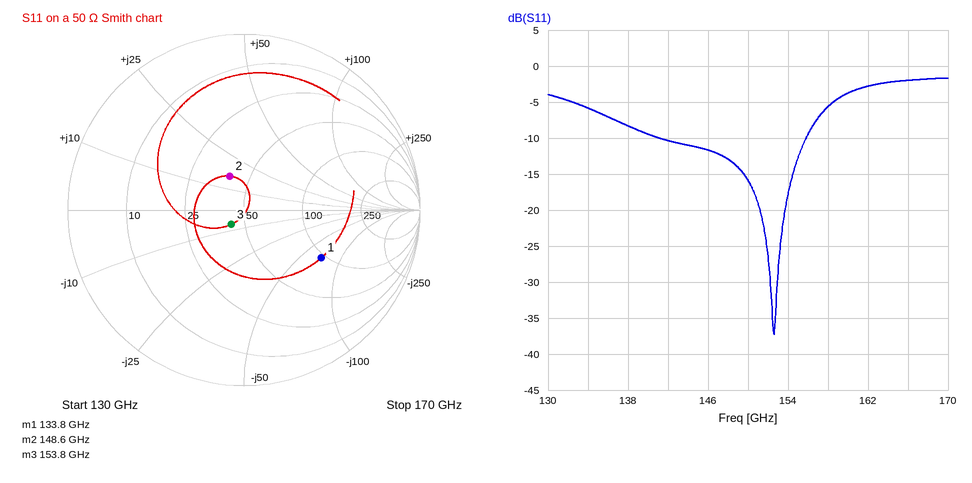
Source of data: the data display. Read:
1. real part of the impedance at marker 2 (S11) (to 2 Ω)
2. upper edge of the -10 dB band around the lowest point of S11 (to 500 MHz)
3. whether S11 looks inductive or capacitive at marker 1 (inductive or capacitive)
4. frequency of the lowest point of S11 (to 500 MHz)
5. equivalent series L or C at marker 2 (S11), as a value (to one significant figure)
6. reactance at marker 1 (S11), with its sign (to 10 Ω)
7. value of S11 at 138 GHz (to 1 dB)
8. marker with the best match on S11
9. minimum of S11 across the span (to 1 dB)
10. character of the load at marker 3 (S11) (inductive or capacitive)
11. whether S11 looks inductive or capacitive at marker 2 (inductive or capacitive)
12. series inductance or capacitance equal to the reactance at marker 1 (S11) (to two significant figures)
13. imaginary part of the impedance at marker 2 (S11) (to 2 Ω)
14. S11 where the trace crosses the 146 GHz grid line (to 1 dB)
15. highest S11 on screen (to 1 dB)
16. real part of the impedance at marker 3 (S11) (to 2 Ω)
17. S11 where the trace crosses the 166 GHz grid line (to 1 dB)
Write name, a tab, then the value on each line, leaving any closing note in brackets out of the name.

real part of the impedance at marker 2 (S11)	40 Ω
upper edge of the -10 dB band around the lowest point of S11	156.0 GHz
whether S11 looks inductive or capacitive at marker 1	capacitive
frequency of the lowest point of S11	152.5 GHz
equivalent series L or C at marker 2 (S11), as a value	20 pH
reactance at marker 1 (S11), with its sign	-70 Ω
value of S11 at 138 GHz	-8 dB
marker with the best match on S11	marker 3
minimum of S11 across the span	-37 dB
character of the load at marker 3 (S11)	capacitive
whether S11 looks inductive or capacitive at marker 2	inductive
series inductance or capacitance equal to the reactance at marker 1 (S11)	17 fF
imaginary part of the impedance at marker 2 (S11)	+16 Ω
S11 where the trace crosses the 146 GHz grid line	-12 dB
highest S11 on screen	-2 dB
real part of the impedance at marker 3 (S11)	42 Ω
S11 where the trace crosses the 166 GHz grid line	-2 dB
